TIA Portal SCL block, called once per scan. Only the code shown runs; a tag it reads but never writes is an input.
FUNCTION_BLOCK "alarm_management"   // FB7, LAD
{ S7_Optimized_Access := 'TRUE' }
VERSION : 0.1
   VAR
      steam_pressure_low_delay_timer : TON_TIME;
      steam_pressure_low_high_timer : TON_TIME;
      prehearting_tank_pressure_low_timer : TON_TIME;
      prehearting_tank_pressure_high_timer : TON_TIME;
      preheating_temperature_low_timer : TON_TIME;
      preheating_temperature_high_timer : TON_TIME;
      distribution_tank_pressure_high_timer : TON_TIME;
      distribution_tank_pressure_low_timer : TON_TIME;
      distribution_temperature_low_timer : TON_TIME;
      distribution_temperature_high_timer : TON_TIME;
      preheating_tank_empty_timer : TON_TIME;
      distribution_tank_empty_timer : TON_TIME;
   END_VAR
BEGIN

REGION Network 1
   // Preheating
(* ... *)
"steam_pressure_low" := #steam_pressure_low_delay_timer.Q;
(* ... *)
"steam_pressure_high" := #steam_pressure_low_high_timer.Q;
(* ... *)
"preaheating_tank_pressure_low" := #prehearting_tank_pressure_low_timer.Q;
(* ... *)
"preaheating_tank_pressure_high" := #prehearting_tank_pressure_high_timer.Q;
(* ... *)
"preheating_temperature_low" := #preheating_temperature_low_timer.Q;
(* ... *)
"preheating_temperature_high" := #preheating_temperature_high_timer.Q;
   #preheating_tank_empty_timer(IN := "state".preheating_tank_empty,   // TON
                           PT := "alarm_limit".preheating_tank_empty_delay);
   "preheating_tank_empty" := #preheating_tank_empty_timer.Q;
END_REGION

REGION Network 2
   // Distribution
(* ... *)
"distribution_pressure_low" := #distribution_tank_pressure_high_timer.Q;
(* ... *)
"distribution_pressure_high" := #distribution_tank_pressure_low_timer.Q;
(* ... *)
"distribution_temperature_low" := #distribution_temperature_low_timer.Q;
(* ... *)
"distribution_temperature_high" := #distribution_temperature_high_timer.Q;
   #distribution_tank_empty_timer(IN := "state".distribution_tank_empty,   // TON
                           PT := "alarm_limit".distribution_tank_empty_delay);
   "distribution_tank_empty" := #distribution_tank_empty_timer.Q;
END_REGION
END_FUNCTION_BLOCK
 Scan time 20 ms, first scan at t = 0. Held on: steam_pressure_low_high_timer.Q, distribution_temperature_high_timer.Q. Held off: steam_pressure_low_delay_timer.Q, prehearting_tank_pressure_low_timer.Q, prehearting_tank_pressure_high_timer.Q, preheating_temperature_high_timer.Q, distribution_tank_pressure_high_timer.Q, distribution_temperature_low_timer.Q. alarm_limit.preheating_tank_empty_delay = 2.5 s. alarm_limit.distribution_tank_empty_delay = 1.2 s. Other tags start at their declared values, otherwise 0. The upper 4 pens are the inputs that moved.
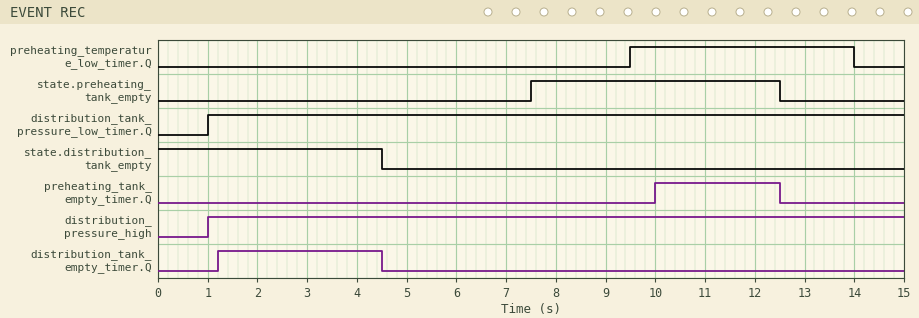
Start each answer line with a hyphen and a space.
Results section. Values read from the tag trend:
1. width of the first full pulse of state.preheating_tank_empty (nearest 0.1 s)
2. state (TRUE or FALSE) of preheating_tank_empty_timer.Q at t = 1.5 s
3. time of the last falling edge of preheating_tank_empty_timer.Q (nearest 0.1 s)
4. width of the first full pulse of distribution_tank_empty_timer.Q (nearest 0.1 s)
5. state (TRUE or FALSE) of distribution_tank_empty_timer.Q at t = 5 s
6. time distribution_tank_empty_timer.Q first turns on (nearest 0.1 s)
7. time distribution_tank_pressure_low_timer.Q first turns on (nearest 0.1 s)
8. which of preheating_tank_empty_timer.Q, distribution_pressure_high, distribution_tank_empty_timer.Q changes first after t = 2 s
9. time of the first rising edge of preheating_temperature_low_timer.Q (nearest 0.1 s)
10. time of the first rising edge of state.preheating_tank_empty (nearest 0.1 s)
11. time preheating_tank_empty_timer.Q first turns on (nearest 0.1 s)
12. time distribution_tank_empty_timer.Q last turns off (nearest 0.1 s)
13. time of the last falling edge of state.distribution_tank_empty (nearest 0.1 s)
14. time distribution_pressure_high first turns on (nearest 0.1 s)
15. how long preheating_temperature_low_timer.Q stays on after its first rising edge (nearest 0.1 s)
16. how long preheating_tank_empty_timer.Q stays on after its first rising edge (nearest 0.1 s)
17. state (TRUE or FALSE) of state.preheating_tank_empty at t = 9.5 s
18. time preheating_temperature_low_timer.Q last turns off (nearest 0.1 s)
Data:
- 5.0 s
- FALSE
- 12.5 s
- 3.3 s
- FALSE
- 1.2 s
- 1.0 s
- distribution_tank_empty_timer.Q
- 9.5 s
- 7.5 s
- 10.0 s
- 4.5 s
- 4.5 s
- 1.0 s
- 4.5 s
- 2.5 s
- TRUE
- 14.0 s
